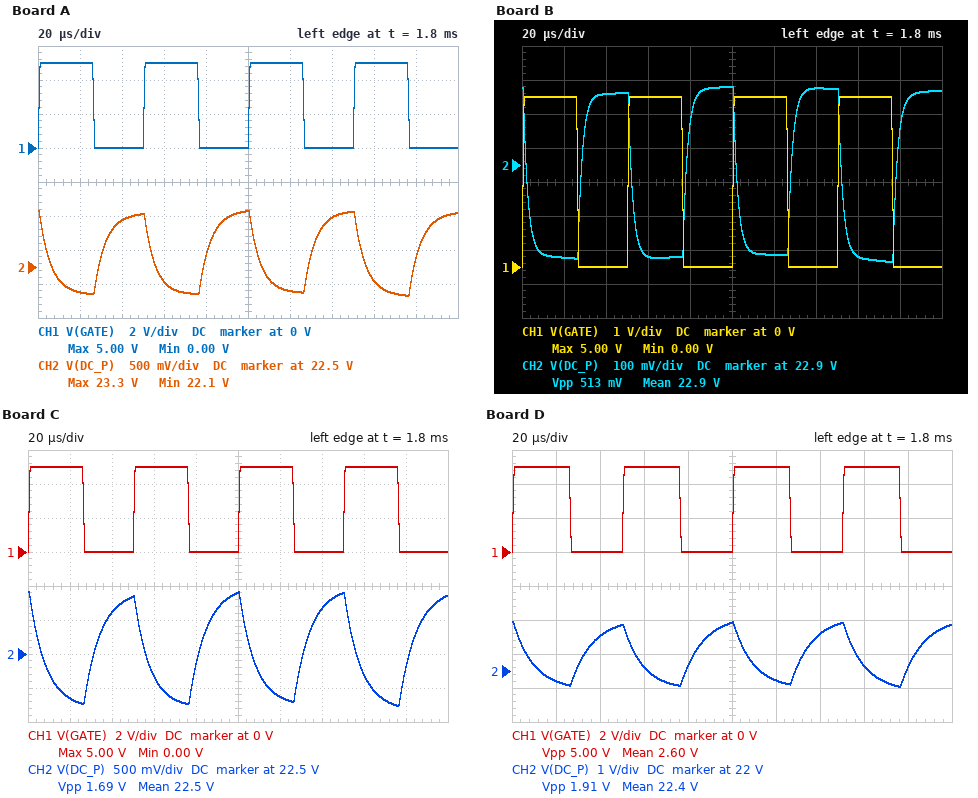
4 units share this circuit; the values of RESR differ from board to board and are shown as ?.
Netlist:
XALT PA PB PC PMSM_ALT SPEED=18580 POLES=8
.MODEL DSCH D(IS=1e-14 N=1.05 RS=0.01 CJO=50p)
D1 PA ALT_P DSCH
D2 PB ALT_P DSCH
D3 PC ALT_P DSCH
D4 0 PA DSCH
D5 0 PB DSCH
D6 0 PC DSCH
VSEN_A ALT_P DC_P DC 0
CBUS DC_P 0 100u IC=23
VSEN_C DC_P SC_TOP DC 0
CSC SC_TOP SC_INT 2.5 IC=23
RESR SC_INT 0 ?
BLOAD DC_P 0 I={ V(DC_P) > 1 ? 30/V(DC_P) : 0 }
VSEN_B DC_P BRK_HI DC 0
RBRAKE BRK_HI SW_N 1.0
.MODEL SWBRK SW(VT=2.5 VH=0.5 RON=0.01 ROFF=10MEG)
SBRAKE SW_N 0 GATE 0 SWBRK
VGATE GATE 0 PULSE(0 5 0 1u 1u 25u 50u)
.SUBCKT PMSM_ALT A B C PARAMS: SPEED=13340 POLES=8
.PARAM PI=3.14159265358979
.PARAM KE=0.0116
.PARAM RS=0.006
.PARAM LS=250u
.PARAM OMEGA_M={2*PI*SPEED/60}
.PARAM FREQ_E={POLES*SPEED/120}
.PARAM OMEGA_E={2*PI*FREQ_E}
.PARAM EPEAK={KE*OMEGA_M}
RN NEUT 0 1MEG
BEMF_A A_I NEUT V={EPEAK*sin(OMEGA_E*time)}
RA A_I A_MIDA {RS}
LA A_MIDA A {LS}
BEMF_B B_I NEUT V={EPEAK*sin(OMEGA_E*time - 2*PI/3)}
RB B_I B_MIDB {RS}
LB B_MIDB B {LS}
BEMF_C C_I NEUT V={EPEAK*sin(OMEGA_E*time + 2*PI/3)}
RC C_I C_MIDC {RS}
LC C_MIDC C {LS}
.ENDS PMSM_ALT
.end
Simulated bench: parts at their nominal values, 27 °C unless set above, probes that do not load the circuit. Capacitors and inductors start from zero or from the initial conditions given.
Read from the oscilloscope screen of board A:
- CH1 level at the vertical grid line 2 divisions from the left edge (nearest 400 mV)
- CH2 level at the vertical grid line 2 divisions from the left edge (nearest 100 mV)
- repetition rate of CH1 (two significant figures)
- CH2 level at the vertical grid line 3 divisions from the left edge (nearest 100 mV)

0 V
23.2 V
20 kHz
22.3 V
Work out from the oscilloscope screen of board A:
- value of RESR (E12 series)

0.056 Ω
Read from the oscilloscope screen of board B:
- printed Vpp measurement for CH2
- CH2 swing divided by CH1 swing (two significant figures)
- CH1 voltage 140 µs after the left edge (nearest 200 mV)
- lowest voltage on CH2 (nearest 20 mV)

513 mV
0.10
0 V
22.62 V
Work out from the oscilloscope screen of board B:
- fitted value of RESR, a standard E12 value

0.022 Ω
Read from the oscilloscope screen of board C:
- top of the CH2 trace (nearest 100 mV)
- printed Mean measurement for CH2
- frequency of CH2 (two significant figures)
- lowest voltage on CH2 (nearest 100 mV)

23.4 V
22.5 V
20 kHz
21.7 V
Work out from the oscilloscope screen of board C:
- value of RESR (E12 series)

0.082 Ω
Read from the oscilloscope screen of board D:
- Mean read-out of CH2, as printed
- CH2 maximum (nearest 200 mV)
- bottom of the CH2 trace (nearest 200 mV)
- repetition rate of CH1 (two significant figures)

22.4 V
23.4 V
21.6 V
20 kHz
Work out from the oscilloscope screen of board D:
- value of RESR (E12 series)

0.1 Ω
